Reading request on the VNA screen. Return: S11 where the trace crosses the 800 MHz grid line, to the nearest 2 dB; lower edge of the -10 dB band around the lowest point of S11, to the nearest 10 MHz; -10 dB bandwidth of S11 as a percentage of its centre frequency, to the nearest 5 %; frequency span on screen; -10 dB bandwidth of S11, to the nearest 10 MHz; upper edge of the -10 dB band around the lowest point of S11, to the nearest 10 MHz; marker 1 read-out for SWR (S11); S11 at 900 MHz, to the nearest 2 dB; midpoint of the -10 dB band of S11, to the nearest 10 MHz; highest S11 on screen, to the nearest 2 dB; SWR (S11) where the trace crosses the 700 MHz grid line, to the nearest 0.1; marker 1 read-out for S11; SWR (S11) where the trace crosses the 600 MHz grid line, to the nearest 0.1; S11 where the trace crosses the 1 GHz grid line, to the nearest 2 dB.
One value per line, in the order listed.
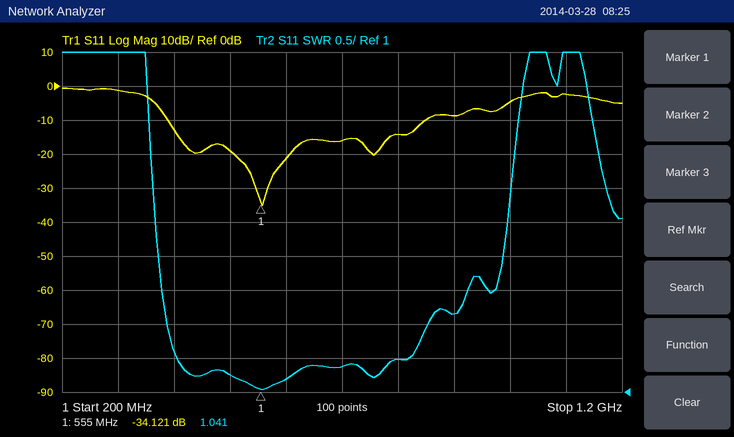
-14 dB
390 MHz
75 %
1 GHz
460 MHz
850 MHz
1.041
-8 dB
620 MHz
0 dB
1.4
-34.121 dB
1.2
-4 dB
